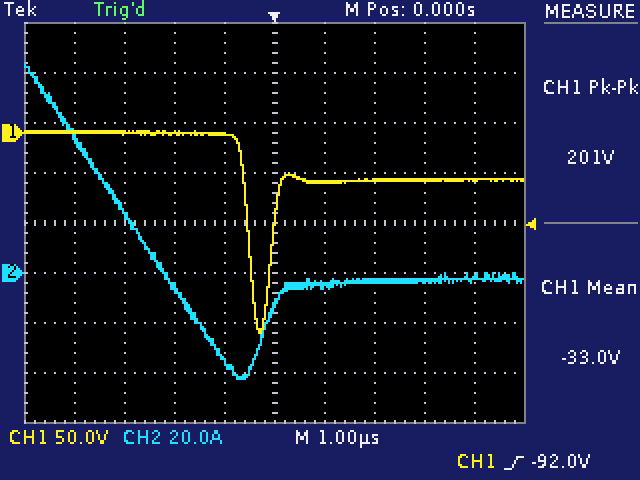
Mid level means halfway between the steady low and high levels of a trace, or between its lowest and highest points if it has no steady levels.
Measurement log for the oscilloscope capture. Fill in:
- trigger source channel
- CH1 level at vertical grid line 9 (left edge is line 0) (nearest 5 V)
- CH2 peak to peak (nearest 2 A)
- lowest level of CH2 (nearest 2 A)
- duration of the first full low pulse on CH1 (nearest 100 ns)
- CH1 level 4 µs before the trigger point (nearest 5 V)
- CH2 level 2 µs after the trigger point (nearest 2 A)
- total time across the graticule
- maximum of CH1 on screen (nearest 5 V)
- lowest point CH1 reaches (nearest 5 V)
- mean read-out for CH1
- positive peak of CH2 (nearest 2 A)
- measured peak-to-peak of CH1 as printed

CH1
-45 V
126 A
-42 A
500 ns
0 V
-4 A
10 µs
0 V
-200 V
-33.0 V
84 A
201 V
